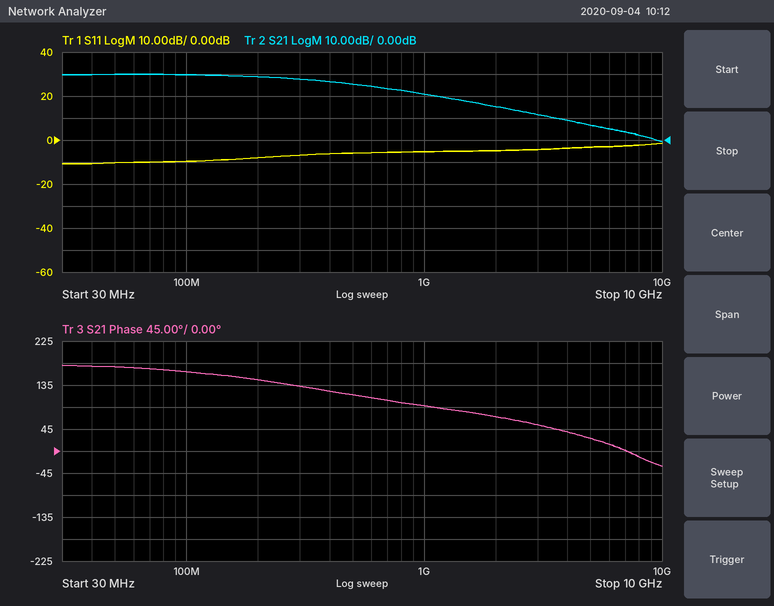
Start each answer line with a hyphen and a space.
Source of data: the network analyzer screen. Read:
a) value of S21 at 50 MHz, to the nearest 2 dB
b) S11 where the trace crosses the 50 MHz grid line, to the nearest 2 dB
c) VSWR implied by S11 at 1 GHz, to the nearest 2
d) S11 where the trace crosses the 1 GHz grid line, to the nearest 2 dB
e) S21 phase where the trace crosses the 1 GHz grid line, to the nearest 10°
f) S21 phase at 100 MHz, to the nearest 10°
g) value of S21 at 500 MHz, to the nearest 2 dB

- 30 dB
- -10 dB
- 4
- -6 dB
- 90°
- 160°
- 26 dB
